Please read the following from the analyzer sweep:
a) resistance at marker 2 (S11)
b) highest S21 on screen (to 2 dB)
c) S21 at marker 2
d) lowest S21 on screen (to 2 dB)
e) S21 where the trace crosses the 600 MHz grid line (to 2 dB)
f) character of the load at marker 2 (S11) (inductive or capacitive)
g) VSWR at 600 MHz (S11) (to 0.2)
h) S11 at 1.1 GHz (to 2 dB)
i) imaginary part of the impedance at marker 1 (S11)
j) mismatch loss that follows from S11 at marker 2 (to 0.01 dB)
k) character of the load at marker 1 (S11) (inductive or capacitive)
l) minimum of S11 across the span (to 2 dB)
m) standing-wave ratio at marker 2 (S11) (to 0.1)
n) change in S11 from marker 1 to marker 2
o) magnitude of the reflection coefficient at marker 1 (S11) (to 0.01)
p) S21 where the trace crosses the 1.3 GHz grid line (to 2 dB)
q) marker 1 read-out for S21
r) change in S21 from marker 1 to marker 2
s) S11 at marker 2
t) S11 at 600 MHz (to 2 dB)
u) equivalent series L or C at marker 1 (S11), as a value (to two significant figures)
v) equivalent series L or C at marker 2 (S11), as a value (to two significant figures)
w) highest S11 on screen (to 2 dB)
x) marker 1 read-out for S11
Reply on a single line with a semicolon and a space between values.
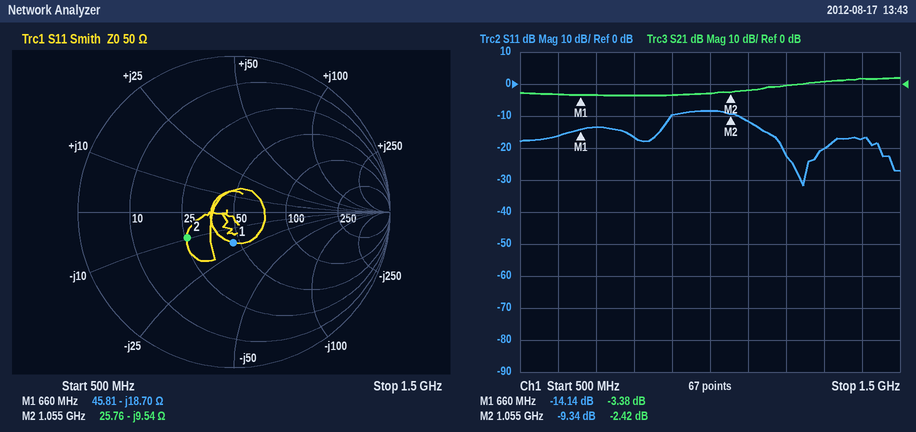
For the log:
25.76 Ω; 2 dB; -2.42 dB; -4 dB; -4 dB; capacitive; 1.4; -12 dB; -18.70 Ω; 0.54 dB; capacitive; -32 dB; 2.0; 4.80 dB; 0.20; 0 dB; -3.38 dB; 0.96 dB; -9.34 dB; -16 dB; 13 pF; 16 pF; -8 dB; -14.14 dB
